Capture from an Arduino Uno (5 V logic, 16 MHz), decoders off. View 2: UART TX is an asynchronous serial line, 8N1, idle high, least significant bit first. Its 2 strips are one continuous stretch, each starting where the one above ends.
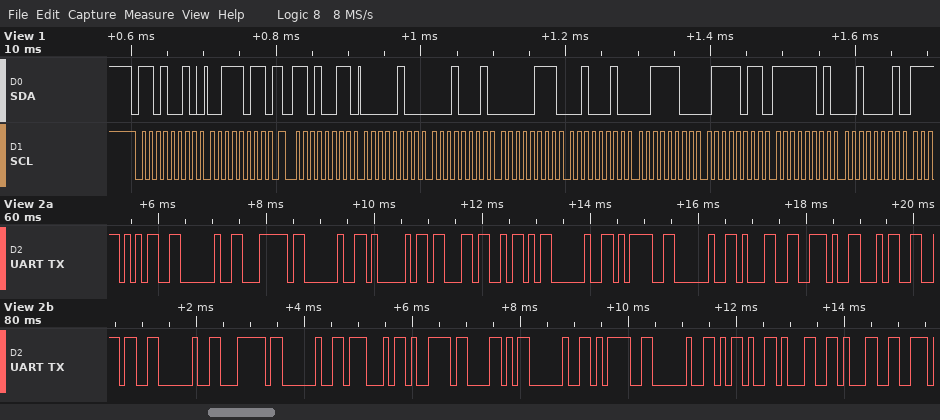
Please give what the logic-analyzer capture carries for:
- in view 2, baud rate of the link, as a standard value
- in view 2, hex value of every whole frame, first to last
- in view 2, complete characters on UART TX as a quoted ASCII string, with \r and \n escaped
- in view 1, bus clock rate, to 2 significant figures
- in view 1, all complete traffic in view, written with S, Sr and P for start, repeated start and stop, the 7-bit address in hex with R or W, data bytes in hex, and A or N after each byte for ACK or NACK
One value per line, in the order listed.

9600 baud
35 20 7C 20 41 63 5A 20 3D 20 31 2E 34 36 20 7C 20 47 79 58 20 3D 20 2D 31 31
"5 | AcZ = 1.46 | GyX = -11"
100 kHz
S 69W A 3B A Sr 69R A 04 A 11 A 07 A 22 A 3C A 7B A FD A 21 A
